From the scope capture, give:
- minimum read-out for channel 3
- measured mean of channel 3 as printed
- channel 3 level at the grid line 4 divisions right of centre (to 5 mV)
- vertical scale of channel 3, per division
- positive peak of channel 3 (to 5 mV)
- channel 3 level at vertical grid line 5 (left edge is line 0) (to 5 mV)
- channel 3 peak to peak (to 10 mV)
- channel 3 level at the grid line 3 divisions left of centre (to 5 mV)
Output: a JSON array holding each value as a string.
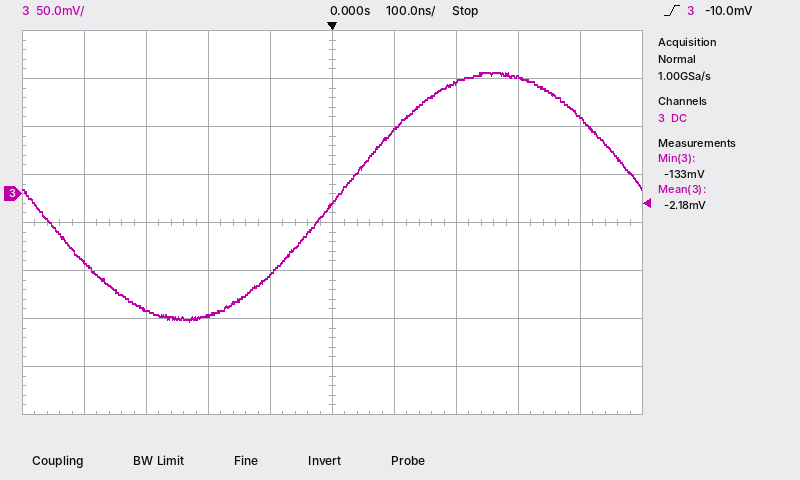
["-133 mV", "-2.18 mV", "80 mV", "50 mV", "125 mV", "-10 mV", "260 mV", "-120 mV"]
